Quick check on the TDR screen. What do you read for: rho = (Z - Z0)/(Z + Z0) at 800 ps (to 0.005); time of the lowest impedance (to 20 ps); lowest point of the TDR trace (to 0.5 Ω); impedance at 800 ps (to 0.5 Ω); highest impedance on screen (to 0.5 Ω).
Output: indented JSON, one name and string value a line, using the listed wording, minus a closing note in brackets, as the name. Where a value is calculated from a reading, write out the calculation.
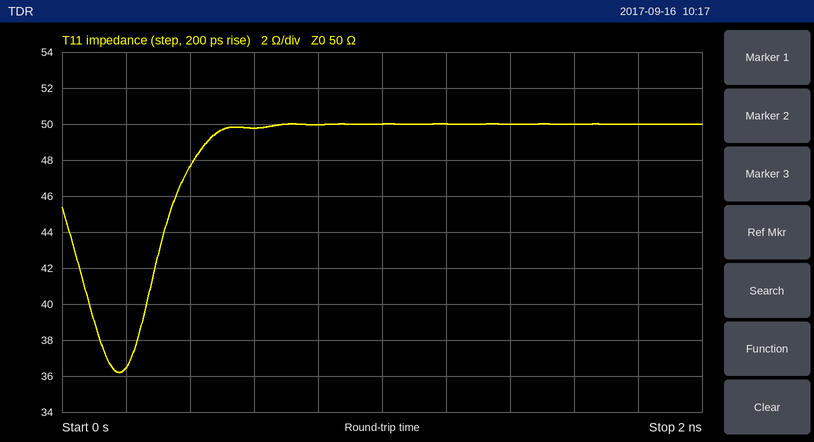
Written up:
{
  "rho = (Z - Z0)/(Z + Z0) at 800 ps": "(50 − 50)/(50 + 50) ≈ 0.000",
  "time of the lowest impedance": "180 ps",
  "lowest point of the TDR trace": "36.0 Ω",
  "impedance at 800 ps": "50.0 Ω",
  "highest impedance on screen": "50.0 Ω"
}
